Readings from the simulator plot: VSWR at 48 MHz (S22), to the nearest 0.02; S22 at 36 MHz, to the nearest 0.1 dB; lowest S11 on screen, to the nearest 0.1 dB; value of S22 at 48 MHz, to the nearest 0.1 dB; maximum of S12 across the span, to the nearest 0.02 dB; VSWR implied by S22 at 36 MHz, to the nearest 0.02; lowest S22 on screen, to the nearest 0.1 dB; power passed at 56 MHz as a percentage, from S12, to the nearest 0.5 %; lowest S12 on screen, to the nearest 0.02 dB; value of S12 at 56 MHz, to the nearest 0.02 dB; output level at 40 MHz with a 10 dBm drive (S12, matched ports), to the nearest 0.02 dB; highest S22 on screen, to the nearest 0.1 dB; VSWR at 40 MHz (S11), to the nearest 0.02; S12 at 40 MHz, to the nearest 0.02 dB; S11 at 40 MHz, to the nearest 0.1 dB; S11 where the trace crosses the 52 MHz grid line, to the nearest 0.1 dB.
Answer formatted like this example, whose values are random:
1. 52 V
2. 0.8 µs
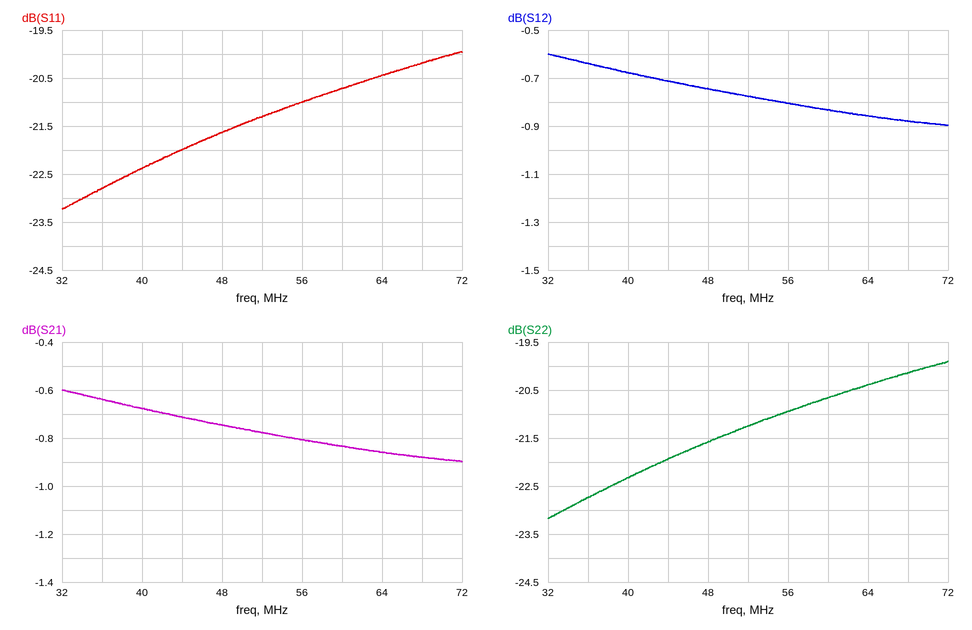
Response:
1. 1.18
2. -22.7 dB
3. -23.2 dB
4. -21.6 dB
5. -0.60 dB
6. 1.16
7. -23.2 dB
8. 83.0 %
9. -0.90 dB
10. -0.80 dB
11. 9.32 dBm
12. -19.9 dB
13. 1.16
14. -0.68 dB
15. -22.4 dB
16. -21.3 dB
